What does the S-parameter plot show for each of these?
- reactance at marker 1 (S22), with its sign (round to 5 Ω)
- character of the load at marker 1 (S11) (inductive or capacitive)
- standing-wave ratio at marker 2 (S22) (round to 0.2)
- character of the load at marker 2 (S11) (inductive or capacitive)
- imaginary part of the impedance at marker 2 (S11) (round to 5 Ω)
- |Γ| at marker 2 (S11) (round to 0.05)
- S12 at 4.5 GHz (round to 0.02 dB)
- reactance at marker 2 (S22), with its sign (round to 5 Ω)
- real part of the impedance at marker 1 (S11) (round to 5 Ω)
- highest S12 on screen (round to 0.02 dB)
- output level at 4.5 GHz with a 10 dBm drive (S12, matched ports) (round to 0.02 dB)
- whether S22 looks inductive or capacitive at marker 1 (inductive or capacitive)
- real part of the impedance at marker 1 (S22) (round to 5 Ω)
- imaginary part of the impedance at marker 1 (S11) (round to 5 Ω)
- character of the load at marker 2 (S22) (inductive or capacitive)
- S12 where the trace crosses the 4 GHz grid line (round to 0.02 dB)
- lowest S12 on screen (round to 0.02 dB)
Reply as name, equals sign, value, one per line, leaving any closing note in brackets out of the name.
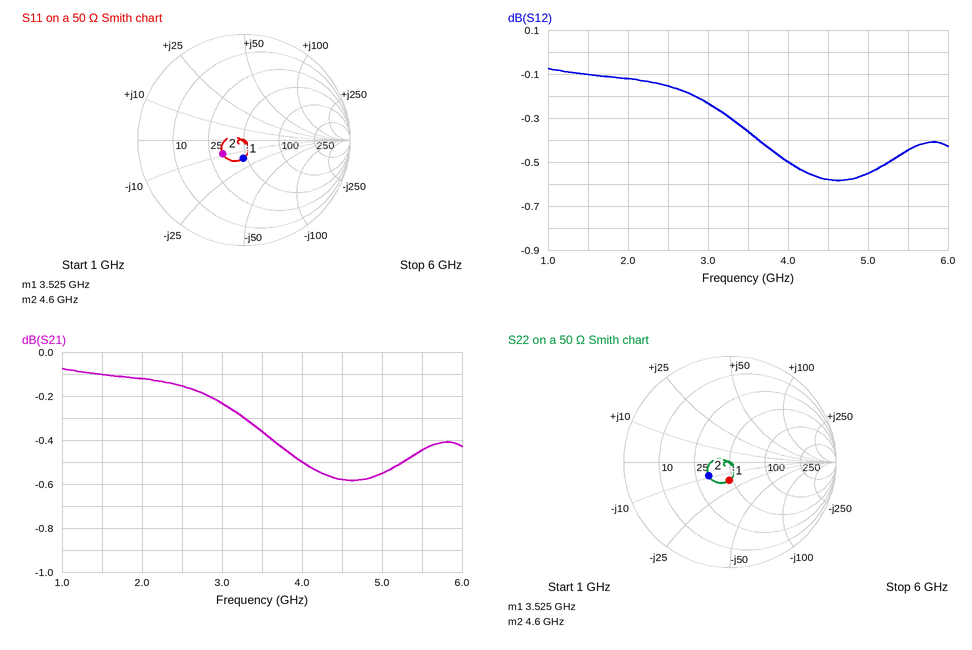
reactance at marker 1 (S22), with its sign = -15 Ω
character of the load at marker 1 (S11) = capacitive
standing-wave ratio at marker 2 (S22) = 1.6
character of the load at marker 2 (S11) = capacitive
imaginary part of the impedance at marker 2 (S11) = -10 Ω
|Γ| at marker 2 (S11) = 0.25
S12 at 4.5 GHz = -0.58 dB
reactance at marker 2 (S22), with its sign = -10 Ω
real part of the impedance at marker 1 (S11) = 45 Ω
highest S12 on screen = -0.08 dB
output level at 4.5 GHz with a 10 dBm drive (S12, matched ports) = 9.42 dBm
whether S22 looks inductive or capacitive at marker 1 = capacitive
real part of the impedance at marker 1 (S22) = 45 Ω
imaginary part of the impedance at marker 1 (S11) = -15 Ω
character of the load at marker 2 (S22) = capacitive
S12 where the trace crosses the 4 GHz grid line = -0.50 dB
lowest S12 on screen = -0.58 dB
